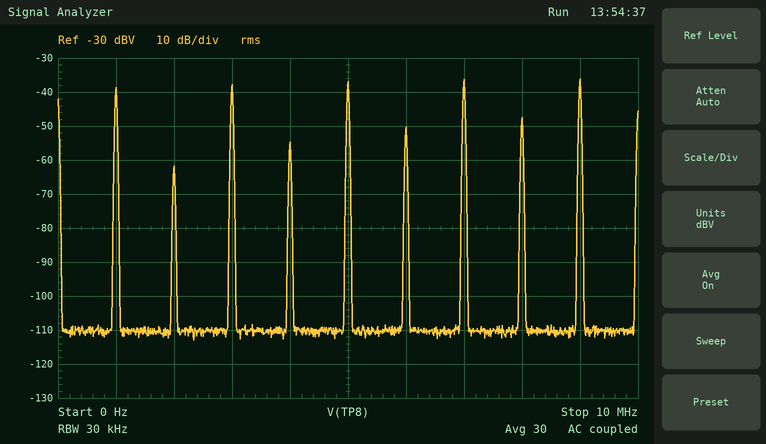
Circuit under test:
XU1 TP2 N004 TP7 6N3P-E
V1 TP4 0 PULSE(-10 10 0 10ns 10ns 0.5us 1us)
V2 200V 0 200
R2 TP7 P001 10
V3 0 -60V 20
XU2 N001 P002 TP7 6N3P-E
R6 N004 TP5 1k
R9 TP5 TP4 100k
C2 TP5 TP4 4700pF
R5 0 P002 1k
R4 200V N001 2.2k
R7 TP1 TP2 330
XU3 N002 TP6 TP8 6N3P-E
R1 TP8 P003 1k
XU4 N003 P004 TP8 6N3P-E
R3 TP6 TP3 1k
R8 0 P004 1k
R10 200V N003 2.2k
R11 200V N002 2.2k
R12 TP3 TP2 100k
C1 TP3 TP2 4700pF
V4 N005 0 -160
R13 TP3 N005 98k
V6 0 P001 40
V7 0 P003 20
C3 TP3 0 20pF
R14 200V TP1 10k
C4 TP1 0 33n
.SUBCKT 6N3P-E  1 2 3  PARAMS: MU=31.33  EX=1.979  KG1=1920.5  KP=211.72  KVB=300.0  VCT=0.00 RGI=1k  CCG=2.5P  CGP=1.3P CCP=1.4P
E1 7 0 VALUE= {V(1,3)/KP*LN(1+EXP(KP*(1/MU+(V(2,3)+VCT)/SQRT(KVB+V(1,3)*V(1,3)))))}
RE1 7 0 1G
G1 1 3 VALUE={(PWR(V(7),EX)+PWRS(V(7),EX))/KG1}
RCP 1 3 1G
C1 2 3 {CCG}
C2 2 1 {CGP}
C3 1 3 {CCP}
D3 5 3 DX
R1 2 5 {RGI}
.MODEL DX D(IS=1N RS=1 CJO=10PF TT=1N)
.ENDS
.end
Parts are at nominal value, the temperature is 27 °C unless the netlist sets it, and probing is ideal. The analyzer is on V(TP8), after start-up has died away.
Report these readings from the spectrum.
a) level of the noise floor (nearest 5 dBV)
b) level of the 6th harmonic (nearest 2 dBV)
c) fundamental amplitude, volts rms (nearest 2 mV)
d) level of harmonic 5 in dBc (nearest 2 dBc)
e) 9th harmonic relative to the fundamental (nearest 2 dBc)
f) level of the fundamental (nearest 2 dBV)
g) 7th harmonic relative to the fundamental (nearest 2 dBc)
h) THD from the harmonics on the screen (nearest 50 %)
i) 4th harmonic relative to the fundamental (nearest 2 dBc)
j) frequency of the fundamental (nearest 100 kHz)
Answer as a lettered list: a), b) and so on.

a) -110 dBV
b) -50 dBV
c) 12 mV
d) 2 dBc
e) 2 dBc
f) -38 dBV
g) 2 dBc
h) 250 %
i) -16 dBc
j) 1.0 MHz
